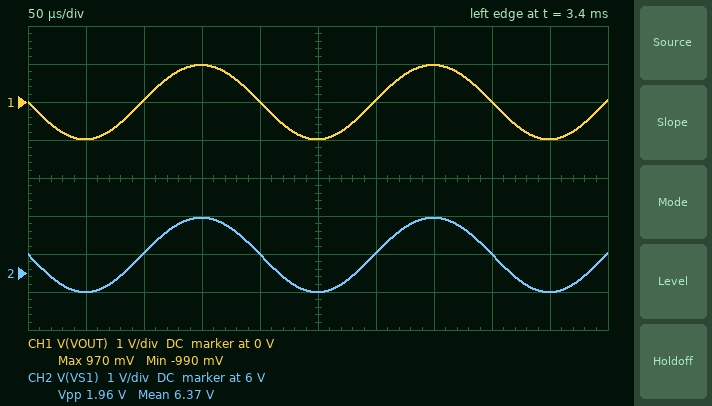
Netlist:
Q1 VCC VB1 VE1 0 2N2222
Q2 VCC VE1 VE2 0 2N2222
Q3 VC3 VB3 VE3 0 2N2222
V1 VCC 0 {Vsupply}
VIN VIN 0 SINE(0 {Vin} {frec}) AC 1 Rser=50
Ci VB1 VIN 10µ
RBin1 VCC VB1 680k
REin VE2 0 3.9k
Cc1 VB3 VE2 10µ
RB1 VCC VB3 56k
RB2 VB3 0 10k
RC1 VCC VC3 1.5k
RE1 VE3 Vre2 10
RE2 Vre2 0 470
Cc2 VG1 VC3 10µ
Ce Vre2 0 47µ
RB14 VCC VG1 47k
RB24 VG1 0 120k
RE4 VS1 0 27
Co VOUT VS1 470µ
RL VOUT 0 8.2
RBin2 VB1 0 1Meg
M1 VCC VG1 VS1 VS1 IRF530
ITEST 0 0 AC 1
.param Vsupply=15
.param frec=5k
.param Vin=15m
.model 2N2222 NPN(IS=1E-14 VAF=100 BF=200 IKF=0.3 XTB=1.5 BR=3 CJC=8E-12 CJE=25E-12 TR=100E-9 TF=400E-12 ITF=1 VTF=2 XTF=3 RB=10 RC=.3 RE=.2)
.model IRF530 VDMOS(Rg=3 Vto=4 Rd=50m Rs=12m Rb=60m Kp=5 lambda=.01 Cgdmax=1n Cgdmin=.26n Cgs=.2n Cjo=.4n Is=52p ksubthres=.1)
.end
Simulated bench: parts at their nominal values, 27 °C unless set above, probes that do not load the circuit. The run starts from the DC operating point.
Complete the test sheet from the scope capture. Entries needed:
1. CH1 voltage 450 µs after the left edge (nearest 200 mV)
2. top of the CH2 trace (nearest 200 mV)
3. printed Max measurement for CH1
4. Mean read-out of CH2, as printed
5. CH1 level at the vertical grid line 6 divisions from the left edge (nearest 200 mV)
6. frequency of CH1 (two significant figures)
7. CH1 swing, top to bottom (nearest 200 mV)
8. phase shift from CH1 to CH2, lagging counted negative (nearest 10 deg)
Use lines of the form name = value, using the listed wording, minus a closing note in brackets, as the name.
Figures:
CH1 voltage 450 µs after the left edge = -1.0 V
top of the CH2 trace = 7.4 V
printed Max measurement for CH1 = 970 mV
Mean read-out of CH2, as printed = 6.37 V
CH1 level at the vertical grid line 6 divisions from the left edge = 0 V
frequency of CH1 = 5.0 kHz
CH1 swing, top to bottom = 2.0 V
phase shift from CH1 to CH2, lagging counted negative = 0 deg
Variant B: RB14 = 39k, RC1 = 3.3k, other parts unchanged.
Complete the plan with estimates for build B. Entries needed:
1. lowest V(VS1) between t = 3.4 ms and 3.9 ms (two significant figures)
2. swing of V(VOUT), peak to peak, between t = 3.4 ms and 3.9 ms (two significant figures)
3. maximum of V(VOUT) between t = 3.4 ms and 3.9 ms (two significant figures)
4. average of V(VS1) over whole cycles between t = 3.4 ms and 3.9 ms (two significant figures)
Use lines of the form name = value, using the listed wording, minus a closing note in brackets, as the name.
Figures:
lowest V(VS1) between t = 3.4 ms and 3.9 ms = 5.4 V
swing of V(VOUT), peak to peak, between t = 3.4 ms and 3.9 ms = 3.6 V
maximum of V(VOUT) between t = 3.4 ms and 3.9 ms = 1.9 V
average of V(VS1) over whole cycles between t = 3.4 ms and 3.9 ms = 7.1 V
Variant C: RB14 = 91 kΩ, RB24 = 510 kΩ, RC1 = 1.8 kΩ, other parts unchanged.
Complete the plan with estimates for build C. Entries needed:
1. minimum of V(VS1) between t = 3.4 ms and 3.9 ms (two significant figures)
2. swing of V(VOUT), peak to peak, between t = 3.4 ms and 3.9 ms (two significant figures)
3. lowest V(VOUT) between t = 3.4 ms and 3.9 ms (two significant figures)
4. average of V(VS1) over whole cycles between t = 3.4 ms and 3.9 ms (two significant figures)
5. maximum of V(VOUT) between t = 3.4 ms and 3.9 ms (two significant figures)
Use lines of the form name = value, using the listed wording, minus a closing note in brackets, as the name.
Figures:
minimum of V(VS1) between t = 3.4 ms and 3.9 ms = 7.2 V
swing of V(VOUT), peak to peak, between t = 3.4 ms and 3.9 ms = 2.4 V
lowest V(VOUT) between t = 3.4 ms and 3.9 ms = -1.2 V
average of V(VS1) over whole cycles between t = 3.4 ms and 3.9 ms = 8.4 V
maximum of V(VOUT) between t = 3.4 ms and 3.9 ms = 1.2 V
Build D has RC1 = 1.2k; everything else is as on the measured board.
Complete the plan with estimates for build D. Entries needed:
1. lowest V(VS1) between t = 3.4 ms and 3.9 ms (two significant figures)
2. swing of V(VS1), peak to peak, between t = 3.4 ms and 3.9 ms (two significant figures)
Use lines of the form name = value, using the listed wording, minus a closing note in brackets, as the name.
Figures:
lowest V(VS1) between t = 3.4 ms and 3.9 ms = 5.7 V
swing of V(VS1), peak to peak, between t = 3.4 ms and 3.9 ms = 1.6 V
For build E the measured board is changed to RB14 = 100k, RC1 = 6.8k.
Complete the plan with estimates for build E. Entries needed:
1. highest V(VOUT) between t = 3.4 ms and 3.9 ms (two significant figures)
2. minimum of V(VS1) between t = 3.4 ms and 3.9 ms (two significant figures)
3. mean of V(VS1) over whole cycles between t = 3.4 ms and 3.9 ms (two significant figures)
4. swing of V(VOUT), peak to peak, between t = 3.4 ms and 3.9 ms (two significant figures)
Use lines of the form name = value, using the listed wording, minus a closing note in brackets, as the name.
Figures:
highest V(VOUT) between t = 3.4 ms and 3.9 ms = 1.9 V
minimum of V(VS1) between t = 3.4 ms and 3.9 ms = 4.0 V
mean of V(VS1) over whole cycles between t = 3.4 ms and 3.9 ms = 4.6 V
swing of V(VOUT), peak to peak, between t = 3.4 ms and 3.9 ms = 2.3 V
